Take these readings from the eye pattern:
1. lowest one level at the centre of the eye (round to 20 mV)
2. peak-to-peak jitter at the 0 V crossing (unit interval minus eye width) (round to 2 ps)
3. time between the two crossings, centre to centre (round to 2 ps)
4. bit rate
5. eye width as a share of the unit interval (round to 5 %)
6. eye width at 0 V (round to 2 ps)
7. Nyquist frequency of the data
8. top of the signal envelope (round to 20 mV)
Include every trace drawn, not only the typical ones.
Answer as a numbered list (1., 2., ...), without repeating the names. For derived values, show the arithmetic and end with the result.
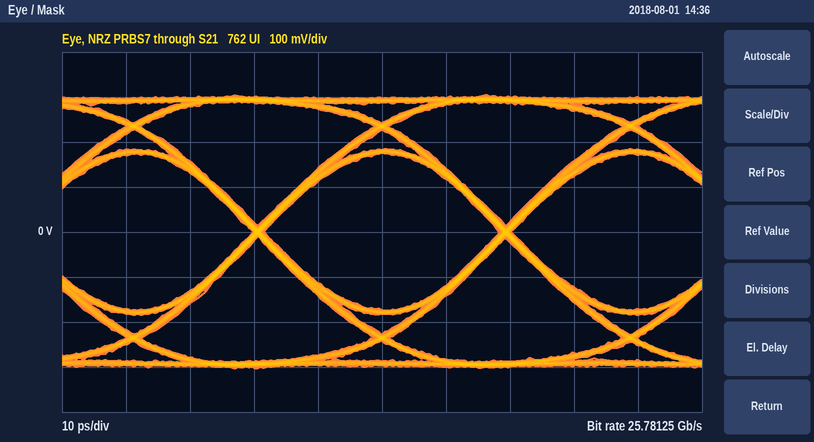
1. 180 mV
2. 2 ps
3. 38 ps
4. 25.78125 Gb/s
5. 36 ps / 38 ps ≈ 95 %
6. 36 ps
7. 12.89062 GHz
8. 300 mV
